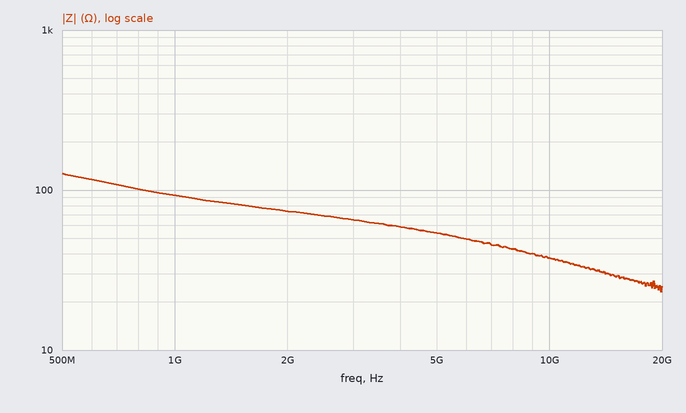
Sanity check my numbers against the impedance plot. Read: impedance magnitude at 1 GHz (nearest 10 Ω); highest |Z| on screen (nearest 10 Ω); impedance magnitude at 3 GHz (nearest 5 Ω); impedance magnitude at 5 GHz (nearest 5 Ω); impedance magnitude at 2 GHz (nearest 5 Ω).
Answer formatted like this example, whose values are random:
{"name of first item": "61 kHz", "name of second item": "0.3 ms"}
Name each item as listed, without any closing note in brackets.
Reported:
{"impedance magnitude at 1 GHz": "90 Ω", "highest |Z| on screen": "130 Ω", "impedance magnitude at 3 GHz": "65 Ω", "impedance magnitude at 5 GHz": "55 Ω", "impedance magnitude at 2 GHz": "75 Ω"}
